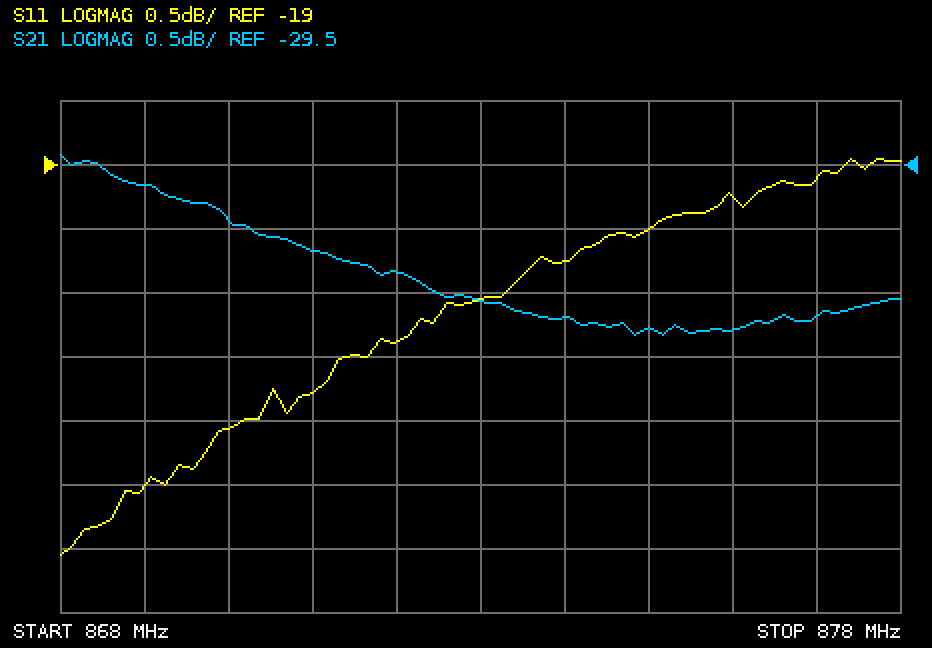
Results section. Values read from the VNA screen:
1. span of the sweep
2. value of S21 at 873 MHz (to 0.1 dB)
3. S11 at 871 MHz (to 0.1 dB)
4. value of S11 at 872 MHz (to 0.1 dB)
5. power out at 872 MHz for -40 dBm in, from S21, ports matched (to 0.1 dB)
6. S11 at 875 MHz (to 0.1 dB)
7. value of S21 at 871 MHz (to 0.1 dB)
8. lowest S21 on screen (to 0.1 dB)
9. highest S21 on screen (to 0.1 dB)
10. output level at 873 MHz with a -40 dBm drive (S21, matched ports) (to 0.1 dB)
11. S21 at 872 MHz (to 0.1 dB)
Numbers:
10 MHz
-30.6 dB
-20.8 dB
-20.4 dB
-70.3 dBm
-19.5 dB
-30.2 dB
-30.8 dB
-29.4 dB
-70.6 dBm
-30.3 dB
